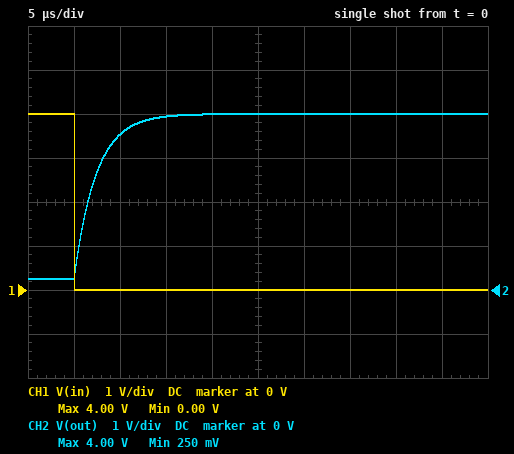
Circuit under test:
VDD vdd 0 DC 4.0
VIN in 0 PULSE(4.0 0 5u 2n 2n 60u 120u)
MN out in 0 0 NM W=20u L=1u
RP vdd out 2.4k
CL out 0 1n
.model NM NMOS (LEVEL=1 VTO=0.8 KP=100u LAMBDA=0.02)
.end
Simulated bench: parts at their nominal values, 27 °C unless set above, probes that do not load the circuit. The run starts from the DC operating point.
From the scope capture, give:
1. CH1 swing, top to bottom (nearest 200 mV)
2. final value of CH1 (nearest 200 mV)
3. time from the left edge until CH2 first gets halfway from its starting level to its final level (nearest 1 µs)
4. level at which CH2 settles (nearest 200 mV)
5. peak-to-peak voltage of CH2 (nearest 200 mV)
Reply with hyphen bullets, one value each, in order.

- 4.0 V
- 0 V
- 7 µs
- 4.0 V
- 3.8 V
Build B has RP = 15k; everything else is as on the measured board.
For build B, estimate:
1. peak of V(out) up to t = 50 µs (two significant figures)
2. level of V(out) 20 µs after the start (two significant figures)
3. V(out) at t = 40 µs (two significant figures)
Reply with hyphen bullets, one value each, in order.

- 3.8 V
- 2.5 V
- 3.6 V
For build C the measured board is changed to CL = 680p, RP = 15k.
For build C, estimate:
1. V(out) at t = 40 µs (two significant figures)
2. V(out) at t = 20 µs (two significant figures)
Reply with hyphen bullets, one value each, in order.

- 3.9 V
- 3.1 V
